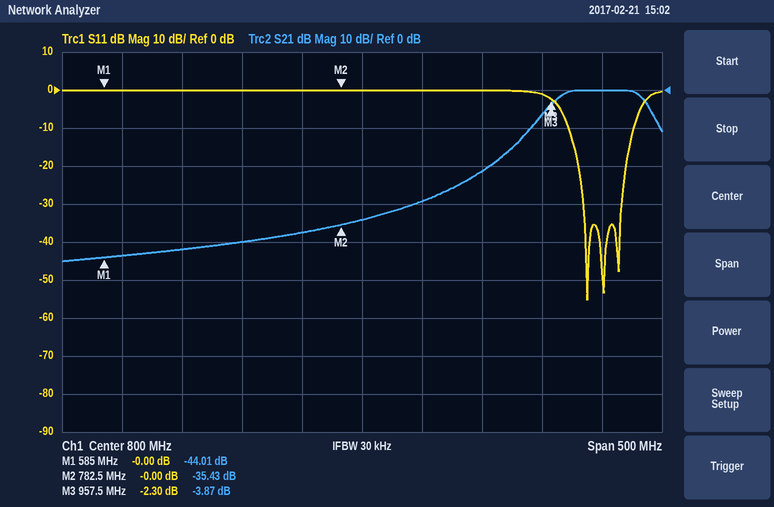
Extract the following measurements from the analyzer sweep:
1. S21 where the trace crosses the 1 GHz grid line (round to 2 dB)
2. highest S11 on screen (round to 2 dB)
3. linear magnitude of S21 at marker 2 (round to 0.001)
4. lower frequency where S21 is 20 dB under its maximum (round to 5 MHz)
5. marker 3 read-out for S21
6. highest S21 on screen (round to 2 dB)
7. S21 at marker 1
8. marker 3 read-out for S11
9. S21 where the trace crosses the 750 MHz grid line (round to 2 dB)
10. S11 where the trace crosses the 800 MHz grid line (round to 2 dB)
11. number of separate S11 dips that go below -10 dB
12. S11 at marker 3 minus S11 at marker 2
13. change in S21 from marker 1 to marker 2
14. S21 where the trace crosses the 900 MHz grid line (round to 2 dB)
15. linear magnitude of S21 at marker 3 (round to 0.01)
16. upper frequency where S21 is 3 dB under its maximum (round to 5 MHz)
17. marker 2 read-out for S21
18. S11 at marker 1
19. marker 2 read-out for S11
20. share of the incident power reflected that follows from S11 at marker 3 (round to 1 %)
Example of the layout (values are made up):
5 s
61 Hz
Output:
0 dB
0 dB
0.017
905 MHz
-3.87 dB
0 dB
-44.01 dB
-2.30 dB
-38 dB
0 dB
3
-2.30 dB
8.58 dB
-22 dB
0.64
1.035 GHz
-35.43 dB
-0.00 dB
-0.00 dB
59 %
